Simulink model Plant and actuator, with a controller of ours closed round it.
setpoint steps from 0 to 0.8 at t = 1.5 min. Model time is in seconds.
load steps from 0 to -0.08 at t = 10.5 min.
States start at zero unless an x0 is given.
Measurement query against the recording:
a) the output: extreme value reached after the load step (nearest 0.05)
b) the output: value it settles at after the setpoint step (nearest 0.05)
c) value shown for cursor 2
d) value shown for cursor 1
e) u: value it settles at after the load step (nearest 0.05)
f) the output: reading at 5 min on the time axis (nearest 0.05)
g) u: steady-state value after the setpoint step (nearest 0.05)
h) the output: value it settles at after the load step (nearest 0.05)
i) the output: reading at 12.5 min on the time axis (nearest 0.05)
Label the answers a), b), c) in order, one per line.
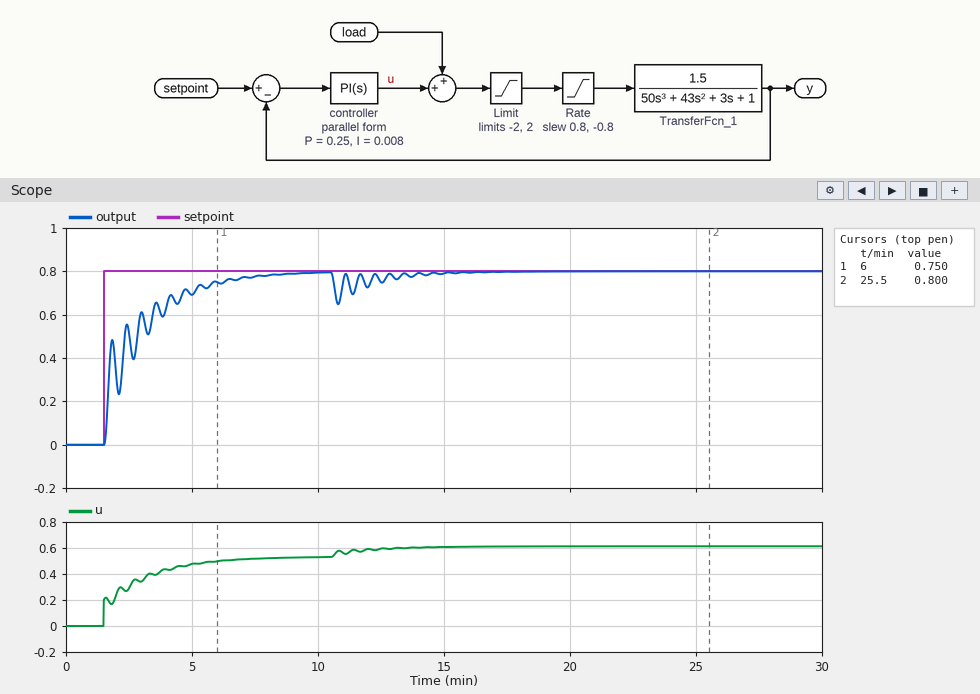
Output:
a) 0.65
b) 0.80
c) 0.800
d) 0.750
e) 0.60
f) 0.70
g) 0.55
h) 0.80
i) 0.75
